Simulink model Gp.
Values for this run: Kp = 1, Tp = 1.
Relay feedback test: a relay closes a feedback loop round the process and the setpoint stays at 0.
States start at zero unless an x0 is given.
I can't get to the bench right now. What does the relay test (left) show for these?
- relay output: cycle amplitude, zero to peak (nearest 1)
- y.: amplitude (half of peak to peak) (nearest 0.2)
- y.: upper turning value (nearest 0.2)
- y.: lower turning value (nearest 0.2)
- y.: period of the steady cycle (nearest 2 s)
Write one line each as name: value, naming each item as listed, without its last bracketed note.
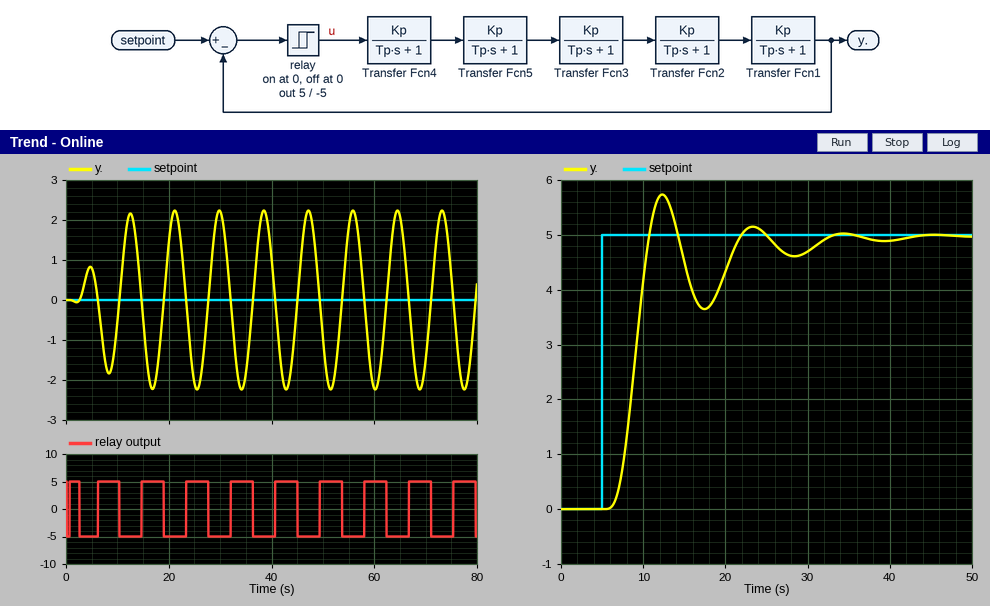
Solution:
relay output: cycle amplitude, zero to peak: 5
y.: amplitude (half of peak to peak): 2.2
y.: upper turning value: 2.2
y.: lower turning value: -2.2
y.: period of the steady cycle: 8 s
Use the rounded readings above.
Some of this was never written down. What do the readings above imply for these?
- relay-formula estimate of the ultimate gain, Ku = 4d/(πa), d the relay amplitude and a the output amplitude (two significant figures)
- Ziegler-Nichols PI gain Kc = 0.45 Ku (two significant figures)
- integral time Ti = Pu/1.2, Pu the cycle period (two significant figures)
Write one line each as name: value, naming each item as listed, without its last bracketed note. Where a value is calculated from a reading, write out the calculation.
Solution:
relay-formula estimate of the ultimate gain, Ku = 4d/(πa), d the relay amplitude and a the output amplitude: 4 × 5 / (π × 2.2) = 2.9
Ziegler-Nichols PI gain Kc = 0.45 Ku: 0.45 × 2.9 = 1.3
integral time Ti = Pu/1.2, Pu the cycle period: 8 / 1.2 = 6.7 s
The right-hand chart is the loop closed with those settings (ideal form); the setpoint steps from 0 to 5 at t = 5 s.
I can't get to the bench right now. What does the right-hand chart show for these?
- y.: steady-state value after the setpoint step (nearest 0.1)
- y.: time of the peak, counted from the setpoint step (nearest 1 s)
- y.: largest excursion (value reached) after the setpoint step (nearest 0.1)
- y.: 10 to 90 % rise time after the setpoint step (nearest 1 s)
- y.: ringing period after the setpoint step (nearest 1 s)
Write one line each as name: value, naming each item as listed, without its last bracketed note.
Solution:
y.: steady-state value after the setpoint step: 5.0
y.: time of the peak, counted from the setpoint step: 7 s
y.: largest excursion (value reached) after the setpoint step: 5.7
y.: 10 to 90 % rise time after the setpoint step: 3 s
y.: ringing period after the setpoint step: 11 s
